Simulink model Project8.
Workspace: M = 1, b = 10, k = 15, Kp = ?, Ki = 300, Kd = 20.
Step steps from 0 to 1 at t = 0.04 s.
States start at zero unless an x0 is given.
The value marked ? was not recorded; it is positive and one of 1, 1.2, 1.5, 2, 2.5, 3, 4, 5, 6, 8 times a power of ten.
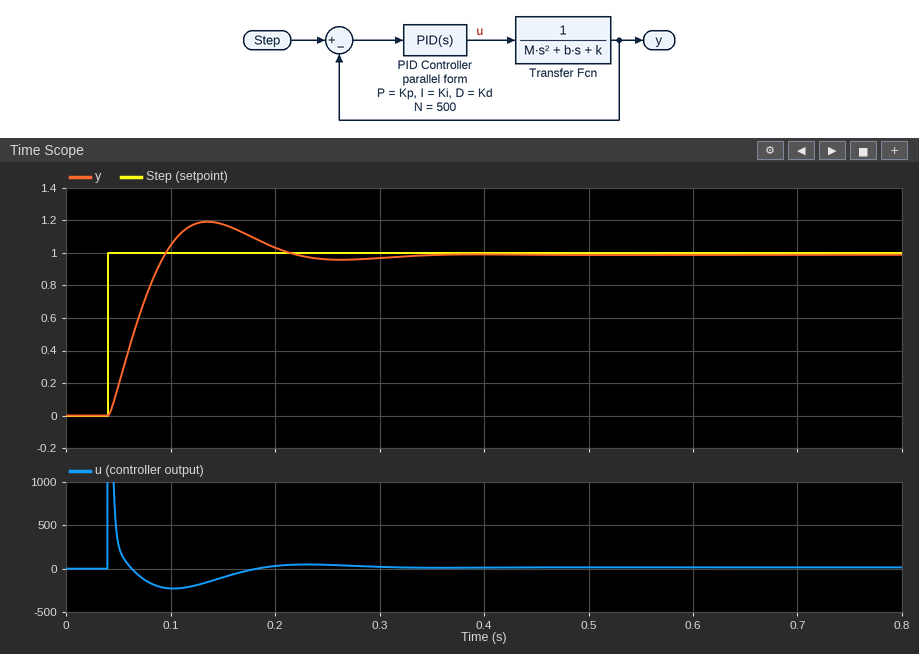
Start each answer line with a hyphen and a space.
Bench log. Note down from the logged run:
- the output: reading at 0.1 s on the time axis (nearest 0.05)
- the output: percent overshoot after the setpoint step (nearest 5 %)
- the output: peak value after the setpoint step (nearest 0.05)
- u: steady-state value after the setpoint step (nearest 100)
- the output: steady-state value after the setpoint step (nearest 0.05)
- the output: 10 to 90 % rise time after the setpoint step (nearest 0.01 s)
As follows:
- 1.05
- 20 %
- 1.20
- 0
- 1.00
- 0.04 s
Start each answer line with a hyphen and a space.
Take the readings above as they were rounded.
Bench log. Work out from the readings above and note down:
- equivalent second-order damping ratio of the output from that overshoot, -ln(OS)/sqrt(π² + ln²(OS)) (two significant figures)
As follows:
- 0.46
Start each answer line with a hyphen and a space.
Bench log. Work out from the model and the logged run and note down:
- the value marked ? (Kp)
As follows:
- 800
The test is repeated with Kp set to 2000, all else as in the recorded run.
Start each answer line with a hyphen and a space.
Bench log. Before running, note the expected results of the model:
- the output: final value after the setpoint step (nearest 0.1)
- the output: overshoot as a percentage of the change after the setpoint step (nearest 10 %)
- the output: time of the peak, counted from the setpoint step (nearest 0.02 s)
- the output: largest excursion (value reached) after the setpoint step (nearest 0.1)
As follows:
- 1.0
- 40 %
- 0.06 s
- 1.4
